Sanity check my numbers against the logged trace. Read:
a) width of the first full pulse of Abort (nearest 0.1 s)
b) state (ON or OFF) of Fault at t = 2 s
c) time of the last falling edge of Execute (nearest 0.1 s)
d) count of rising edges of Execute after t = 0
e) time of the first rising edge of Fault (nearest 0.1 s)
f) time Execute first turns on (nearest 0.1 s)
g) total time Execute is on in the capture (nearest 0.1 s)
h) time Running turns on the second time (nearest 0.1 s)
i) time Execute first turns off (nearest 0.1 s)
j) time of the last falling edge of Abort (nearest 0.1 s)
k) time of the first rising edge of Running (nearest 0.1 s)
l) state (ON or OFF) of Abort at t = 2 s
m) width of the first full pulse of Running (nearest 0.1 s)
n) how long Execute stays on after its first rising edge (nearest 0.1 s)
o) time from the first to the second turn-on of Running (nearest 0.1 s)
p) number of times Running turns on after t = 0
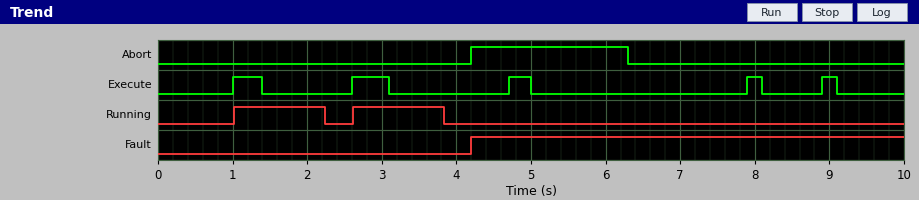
2.1 s
OFF
9.1 s
5
4.2 s
1.0 s
1.6 s
2.6 s
1.4 s
6.3 s
1.0 s
OFF
1.2 s
0.4 s
1.6 s
2
